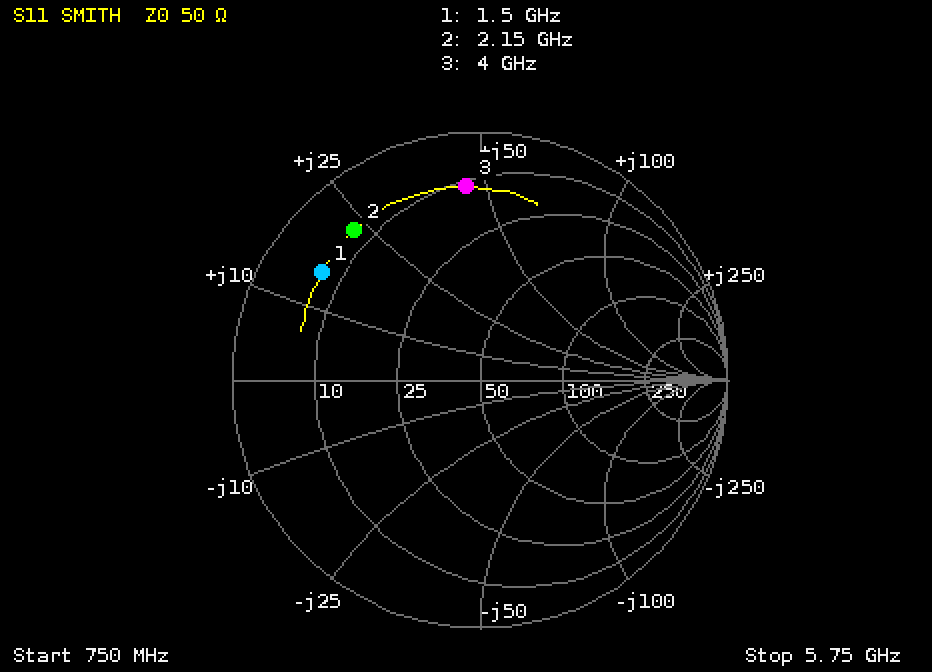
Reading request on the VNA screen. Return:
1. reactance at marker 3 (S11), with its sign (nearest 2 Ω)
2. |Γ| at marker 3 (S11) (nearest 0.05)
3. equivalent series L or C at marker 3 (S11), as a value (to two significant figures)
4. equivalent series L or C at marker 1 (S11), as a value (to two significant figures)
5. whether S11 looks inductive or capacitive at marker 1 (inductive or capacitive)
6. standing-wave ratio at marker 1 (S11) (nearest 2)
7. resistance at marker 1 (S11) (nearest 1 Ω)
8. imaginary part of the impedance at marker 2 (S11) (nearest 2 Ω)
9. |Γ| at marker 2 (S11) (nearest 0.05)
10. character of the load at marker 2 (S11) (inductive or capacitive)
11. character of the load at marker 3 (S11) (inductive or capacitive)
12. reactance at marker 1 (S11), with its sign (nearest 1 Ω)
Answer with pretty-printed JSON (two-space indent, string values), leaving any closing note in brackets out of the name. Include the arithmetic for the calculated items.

{
  "reactance at marker 3 (S11), with its sign": "+46 Ω",
  "|Γ| at marker 3 (S11)": "0.80",
  "equivalent series L or C at marker 3 (S11), as a value": "L = 46 Ω/(2π × 4 GHz) ≈ 1.8 nH",
  "equivalent series L or C at marker 1 (S11), as a value": "L = 15 Ω/(2π × 1.5 GHz) ≈ 1.6 nH",
  "whether S11 looks inductive or capacitive at marker 1": "inductive",
  "standing-wave ratio at marker 1 (S11)": "8",
  "resistance at marker 1 (S11)": "7 Ω",
  "imaginary part of the impedance at marker 2 (S11)": "+22 Ω",
  "|Γ| at marker 2 (S11)": "0.80",
  "character of the load at marker 2 (S11)": "inductive",
  "character of the load at marker 3 (S11)": "inductive",
  "reactance at marker 1 (S11), with its sign": "+15 Ω"
}
